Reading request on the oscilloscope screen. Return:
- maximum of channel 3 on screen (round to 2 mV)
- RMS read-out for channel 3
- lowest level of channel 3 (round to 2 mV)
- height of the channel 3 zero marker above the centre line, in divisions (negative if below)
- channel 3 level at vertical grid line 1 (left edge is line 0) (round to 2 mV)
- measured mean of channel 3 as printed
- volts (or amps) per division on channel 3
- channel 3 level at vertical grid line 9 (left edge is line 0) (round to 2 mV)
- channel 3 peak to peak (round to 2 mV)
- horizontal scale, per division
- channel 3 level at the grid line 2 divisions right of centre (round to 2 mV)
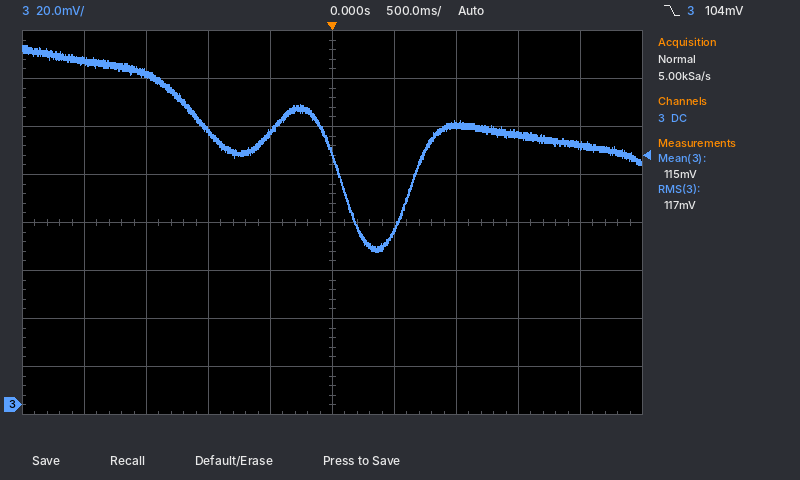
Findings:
150 mV
117 mV
64 mV
-3.8 div
144 mV
115 mV
20 mV
108 mV
86 mV
500 ms
116 mV
